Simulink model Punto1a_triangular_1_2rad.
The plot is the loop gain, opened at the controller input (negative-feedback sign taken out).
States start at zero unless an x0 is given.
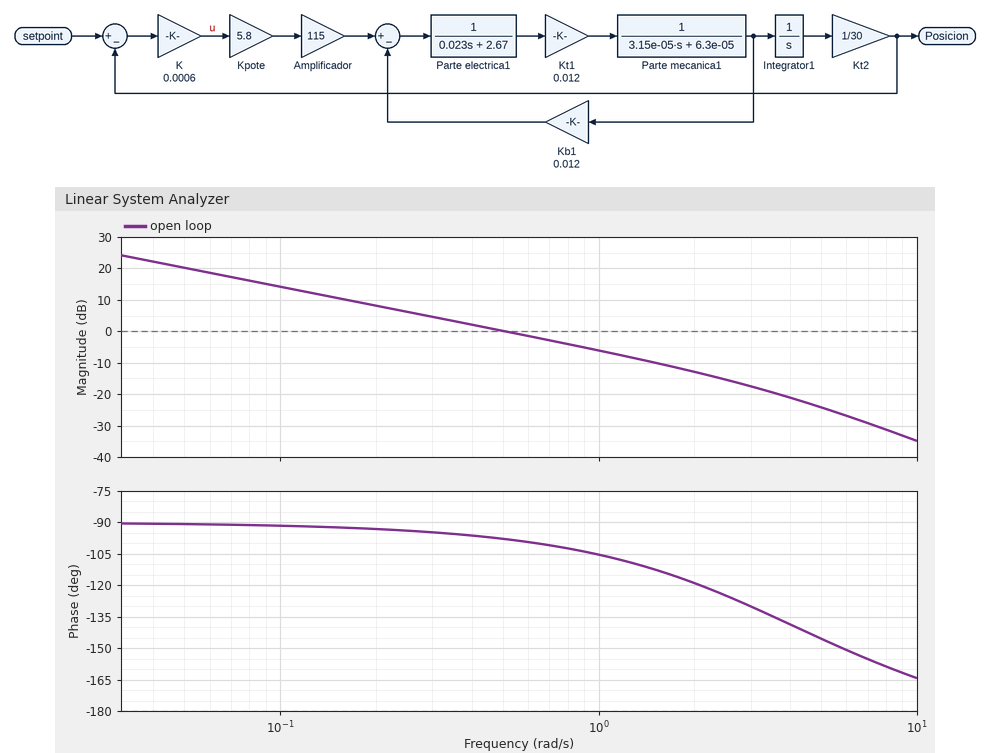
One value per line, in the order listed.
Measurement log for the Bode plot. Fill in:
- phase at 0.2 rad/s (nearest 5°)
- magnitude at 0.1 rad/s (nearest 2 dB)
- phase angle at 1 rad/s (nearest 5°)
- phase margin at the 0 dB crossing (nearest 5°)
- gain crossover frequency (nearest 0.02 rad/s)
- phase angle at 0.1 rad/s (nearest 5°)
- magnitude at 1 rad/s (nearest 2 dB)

-95°
14 dB
-105°
80°
0.50 rad/s
-90°
-6 dB
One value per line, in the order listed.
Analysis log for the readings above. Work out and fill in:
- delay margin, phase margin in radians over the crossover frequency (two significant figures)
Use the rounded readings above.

2.8 s
